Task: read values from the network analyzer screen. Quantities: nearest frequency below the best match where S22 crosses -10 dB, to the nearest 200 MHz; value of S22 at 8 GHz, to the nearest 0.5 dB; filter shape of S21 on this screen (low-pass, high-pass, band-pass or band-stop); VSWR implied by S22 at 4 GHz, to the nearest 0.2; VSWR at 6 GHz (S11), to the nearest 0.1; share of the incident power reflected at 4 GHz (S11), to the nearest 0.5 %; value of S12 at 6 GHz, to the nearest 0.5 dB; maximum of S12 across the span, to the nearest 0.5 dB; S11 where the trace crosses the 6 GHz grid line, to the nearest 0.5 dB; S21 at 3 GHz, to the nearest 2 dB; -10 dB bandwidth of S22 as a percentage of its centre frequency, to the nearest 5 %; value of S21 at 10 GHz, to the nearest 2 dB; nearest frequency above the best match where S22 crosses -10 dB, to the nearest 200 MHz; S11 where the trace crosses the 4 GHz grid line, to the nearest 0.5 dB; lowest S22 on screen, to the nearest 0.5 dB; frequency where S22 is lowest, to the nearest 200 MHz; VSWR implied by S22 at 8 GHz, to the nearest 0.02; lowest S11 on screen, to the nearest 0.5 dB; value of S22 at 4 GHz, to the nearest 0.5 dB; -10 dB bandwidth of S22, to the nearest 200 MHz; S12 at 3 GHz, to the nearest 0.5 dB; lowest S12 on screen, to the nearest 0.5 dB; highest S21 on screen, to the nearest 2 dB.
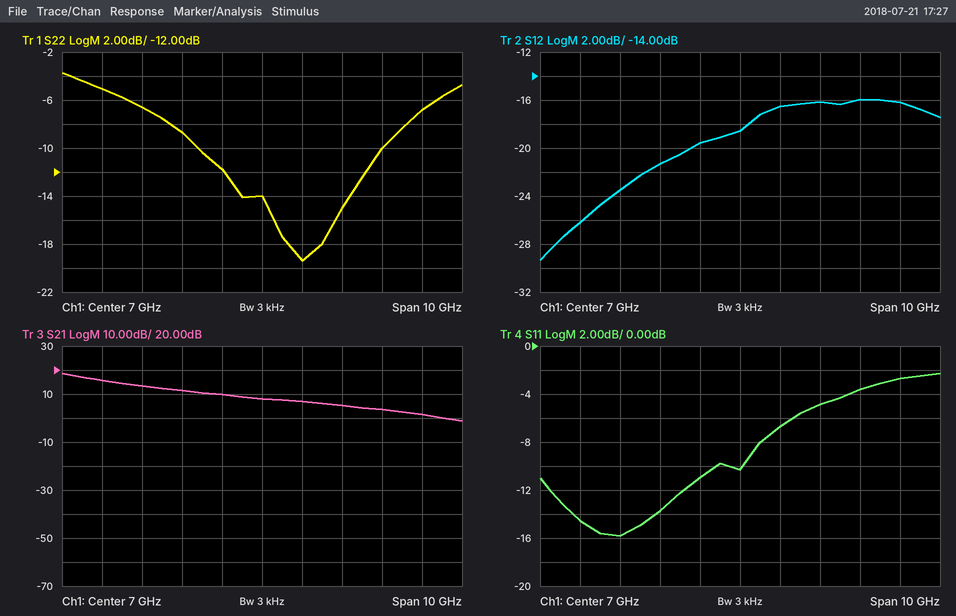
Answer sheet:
5.4 GHz
-19.5 dB
low-pass
2.8
1.8
2.5 %
-19.5 dB
-16.0 dB
-11.0 dB
16 dB
60 %
4 dB
10.0 GHz
-16.0 dB
-19.5 dB
8.0 GHz
1.24
-16.0 dB
-6.5 dB
4.6 GHz
-26.0 dB
-29.5 dB
18 dB
